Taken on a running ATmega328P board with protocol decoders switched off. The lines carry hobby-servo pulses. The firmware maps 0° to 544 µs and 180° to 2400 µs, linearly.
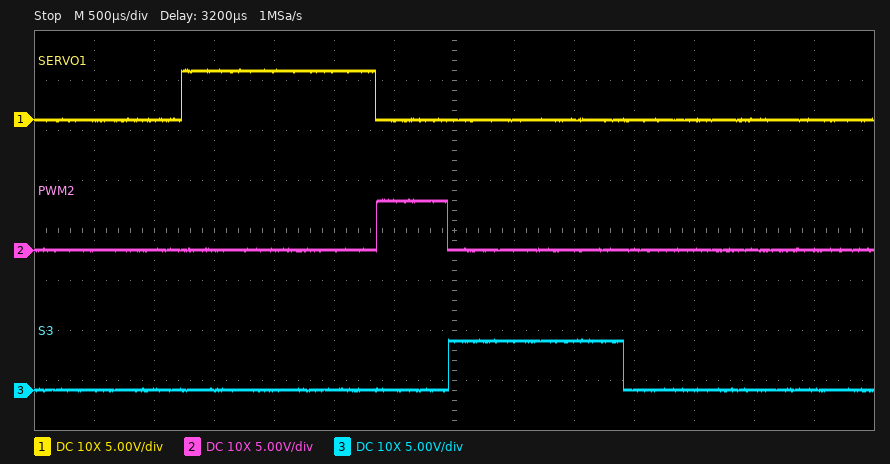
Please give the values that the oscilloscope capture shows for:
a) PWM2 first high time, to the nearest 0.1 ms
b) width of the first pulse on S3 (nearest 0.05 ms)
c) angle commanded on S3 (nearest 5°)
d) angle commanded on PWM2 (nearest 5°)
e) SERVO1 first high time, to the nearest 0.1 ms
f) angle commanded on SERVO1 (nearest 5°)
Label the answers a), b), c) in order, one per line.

a) 0.6 ms
b) 1.45 ms
c) 90°
d) 5°
e) 1.6 ms
f) 105°
